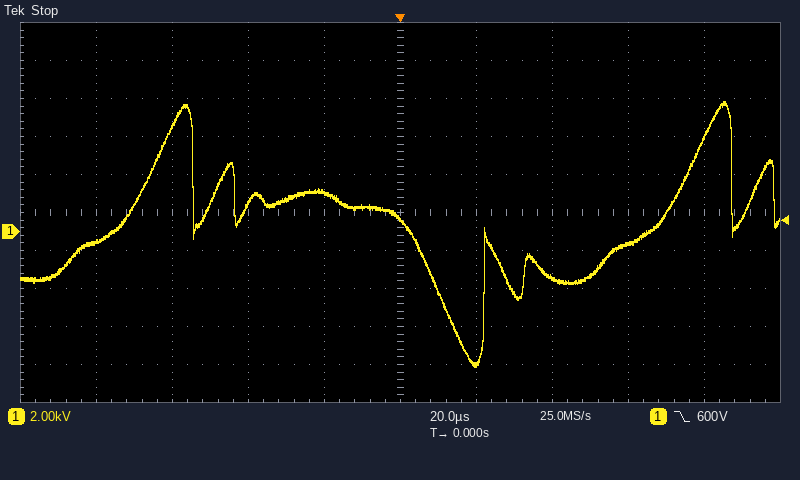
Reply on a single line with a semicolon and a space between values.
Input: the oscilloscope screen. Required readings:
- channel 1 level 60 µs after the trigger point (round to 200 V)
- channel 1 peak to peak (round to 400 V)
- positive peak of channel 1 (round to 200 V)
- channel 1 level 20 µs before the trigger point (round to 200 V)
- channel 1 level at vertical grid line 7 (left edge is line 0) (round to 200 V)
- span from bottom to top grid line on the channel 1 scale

-600 V; 14.0 kV; 6.8 kV; 2.0 kV; -2.4 kV; 20 kV
